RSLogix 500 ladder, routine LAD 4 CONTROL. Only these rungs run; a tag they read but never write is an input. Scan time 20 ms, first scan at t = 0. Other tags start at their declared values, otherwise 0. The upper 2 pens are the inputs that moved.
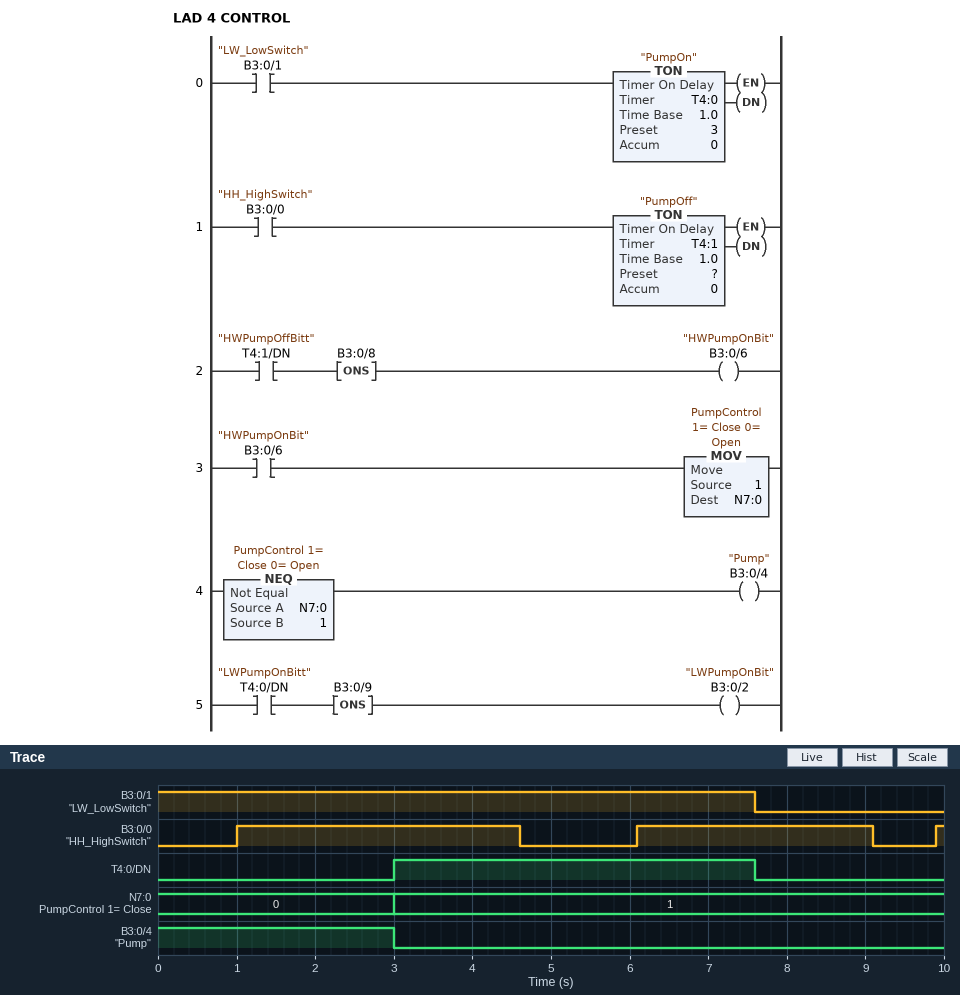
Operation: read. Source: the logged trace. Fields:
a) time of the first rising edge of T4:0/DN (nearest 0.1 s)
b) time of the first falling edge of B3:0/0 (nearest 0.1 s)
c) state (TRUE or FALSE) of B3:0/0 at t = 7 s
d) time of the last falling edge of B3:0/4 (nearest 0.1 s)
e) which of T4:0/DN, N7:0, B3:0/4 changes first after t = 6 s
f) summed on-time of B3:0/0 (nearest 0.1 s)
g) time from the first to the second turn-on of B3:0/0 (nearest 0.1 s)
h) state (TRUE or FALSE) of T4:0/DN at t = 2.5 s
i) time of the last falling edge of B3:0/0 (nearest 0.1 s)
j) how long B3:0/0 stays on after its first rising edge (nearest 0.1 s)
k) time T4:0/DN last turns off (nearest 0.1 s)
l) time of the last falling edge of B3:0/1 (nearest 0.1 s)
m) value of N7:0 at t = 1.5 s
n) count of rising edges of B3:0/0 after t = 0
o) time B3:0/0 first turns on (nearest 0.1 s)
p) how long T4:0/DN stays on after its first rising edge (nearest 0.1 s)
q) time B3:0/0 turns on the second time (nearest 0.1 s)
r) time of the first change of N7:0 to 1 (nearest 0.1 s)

3.0 s
4.6 s
TRUE
3.0 s
T4:0/DN
6.7 s
5.1 s
FALSE
9.1 s
3.6 s
7.6 s
7.6 s
0
3
1.0 s
4.6 s
6.1 s
3.0 s
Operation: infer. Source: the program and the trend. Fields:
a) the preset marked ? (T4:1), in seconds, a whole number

2 s
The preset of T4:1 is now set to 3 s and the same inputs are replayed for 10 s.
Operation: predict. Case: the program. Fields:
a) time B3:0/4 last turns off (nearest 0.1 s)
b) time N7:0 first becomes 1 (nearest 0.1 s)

4.0 s
4.0 s
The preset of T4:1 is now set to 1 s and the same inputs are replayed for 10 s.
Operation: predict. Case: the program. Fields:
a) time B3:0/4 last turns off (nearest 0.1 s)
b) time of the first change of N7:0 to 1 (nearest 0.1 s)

2.0 s
2.0 s
